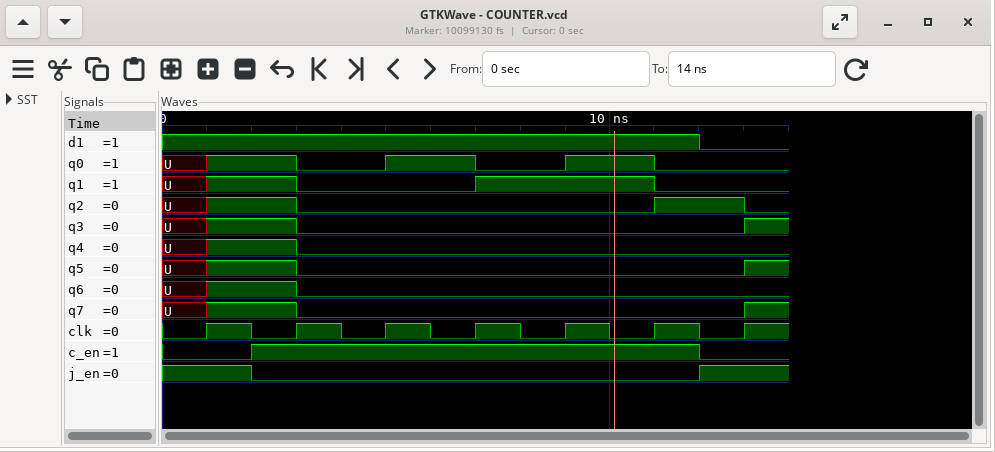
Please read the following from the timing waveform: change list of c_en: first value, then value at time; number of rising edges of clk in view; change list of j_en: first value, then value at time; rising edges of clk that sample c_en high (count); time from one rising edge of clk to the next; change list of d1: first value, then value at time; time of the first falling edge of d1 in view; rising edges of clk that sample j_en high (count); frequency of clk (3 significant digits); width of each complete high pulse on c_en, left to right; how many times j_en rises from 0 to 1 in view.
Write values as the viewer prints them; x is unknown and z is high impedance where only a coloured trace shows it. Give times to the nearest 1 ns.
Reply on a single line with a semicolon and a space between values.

0, 1 at 2 ns, 0 at 12 ns; 7; 1, 0 at 2 ns, 1 at 12 ns; 5; 2 ns; 1, 0 at 12 ns; 12 ns; 2; 500 MHz; 10 ns; 1
